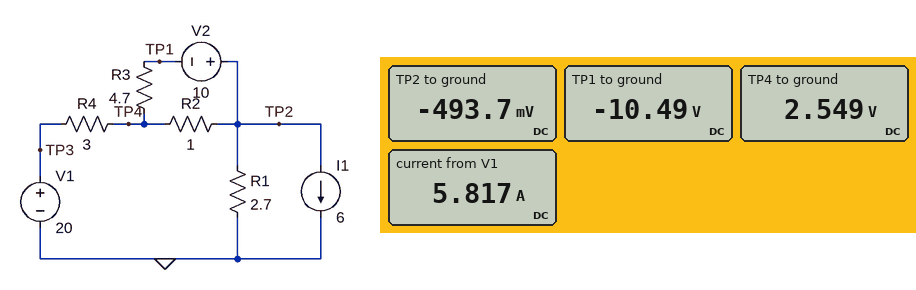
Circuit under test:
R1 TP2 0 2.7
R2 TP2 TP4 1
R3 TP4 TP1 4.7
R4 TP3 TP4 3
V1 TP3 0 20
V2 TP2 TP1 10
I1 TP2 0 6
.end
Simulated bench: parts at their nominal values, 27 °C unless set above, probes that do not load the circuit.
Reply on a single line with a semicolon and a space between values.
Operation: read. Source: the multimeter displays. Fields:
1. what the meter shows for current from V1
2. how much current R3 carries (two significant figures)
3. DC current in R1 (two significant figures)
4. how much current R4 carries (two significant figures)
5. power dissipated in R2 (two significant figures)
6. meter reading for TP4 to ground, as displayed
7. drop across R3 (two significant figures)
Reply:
5.817 A; 2.8 A; 180 mA; 5.8 A; 9.3 W; 2.549 V; 13 V
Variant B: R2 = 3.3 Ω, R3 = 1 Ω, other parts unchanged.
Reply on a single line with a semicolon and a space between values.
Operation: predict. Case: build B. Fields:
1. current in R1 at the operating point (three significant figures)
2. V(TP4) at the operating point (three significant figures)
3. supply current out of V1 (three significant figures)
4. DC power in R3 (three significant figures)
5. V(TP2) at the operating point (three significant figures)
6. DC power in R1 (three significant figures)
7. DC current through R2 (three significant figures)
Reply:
784 mA; -352 mV; 6.78 A; 56.7 W; 2.12 V; 1.66 W; 748 mA
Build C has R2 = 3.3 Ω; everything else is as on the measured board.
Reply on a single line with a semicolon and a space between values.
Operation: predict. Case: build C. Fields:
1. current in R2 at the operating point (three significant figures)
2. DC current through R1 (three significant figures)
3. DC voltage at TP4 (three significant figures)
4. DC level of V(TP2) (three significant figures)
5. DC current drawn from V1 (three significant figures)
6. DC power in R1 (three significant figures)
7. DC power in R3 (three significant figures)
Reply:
1.85 A; 721 mA; 4.16 V; -1.95 V; 5.28 A; 1.40 W; 55.2 W
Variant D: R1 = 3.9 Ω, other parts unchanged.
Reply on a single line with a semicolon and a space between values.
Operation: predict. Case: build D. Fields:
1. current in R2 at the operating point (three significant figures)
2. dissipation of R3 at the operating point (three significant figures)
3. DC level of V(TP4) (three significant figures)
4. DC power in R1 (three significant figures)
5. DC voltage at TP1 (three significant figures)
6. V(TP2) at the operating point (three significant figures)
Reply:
3.07 A; 36.3 W; 2.46 V; 93.0 mW; -10.6 V; -602 mV
